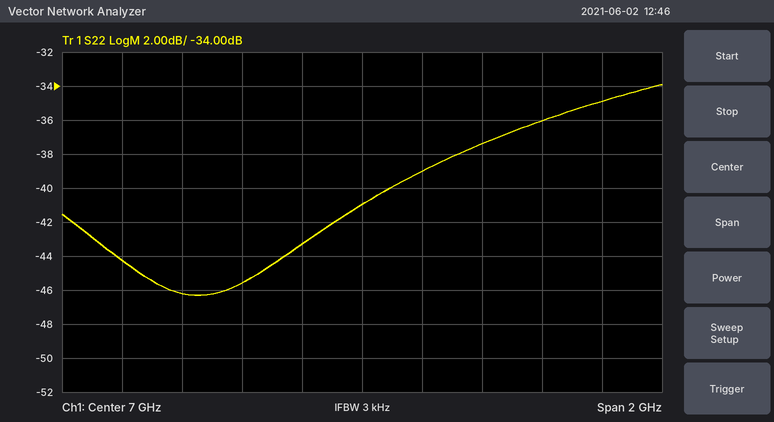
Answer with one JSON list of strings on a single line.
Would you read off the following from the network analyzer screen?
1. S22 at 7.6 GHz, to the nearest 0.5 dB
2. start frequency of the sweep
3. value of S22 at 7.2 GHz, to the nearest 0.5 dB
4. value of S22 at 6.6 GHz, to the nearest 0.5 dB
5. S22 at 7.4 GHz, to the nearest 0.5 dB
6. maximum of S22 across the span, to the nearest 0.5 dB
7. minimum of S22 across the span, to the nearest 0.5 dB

["-36.0 dB", "6 GHz", "-39.0 dB", "-45.5 dB", "-37.5 dB", "-34.0 dB", "-46.5 dB"]
